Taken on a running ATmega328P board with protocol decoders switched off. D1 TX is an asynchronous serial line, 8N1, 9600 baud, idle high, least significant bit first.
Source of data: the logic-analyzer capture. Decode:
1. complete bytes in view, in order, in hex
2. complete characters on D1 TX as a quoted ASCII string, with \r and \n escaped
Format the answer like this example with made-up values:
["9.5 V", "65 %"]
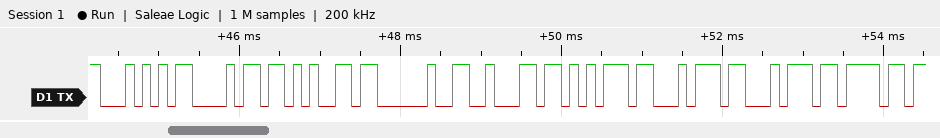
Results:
["0x54 0x68 0x65 0x20 0x62 0x75 0x74 0x74 0x6F", "\"The butto\""]
